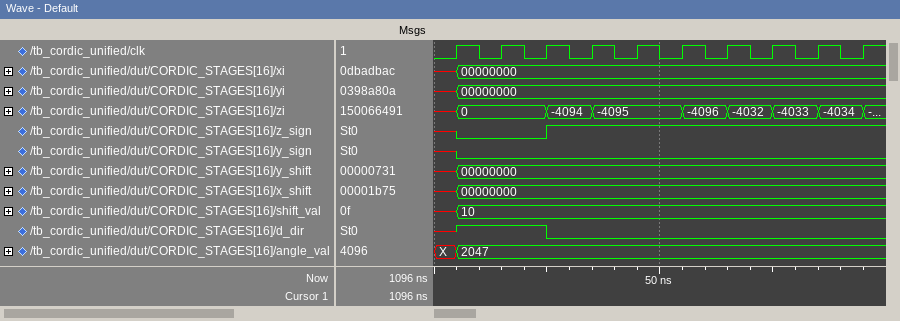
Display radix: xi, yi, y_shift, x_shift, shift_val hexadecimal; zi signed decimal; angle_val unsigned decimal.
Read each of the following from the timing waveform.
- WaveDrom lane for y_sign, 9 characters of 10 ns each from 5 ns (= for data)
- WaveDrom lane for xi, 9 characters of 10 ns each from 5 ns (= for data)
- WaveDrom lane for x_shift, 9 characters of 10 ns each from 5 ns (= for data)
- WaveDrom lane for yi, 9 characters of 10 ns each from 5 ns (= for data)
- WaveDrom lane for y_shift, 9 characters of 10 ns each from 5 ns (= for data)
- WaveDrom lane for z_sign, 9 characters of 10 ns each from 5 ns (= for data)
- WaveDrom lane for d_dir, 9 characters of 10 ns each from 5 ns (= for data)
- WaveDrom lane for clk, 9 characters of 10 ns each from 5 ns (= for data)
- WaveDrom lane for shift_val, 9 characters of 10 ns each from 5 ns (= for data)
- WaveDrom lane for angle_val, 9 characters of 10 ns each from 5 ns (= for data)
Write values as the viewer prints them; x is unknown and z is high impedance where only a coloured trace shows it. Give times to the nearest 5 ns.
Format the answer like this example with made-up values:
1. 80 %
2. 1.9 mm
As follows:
1. {name: 'y_sign', wave: '0........'}
2. {name: 'xi', wave: '=........', data: '00000000'}
3. {name: 'x_shift', wave: '=........', data: '00000000'}
4. {name: 'yi', wave: '=........', data: '00000000'}
5. {name: 'y_shift', wave: '=........', data: '00000000'}
6. {name: 'z_sign', wave: '0.1......'}
7. {name: 'd_dir', wave: '1.0......'}
8. {name: 'clk', wave: 'p........'}
9. {name: 'shift_val', wave: '=........', data: '10'}
10. {name: 'angle_val', wave: '=........', data: '2047'}
